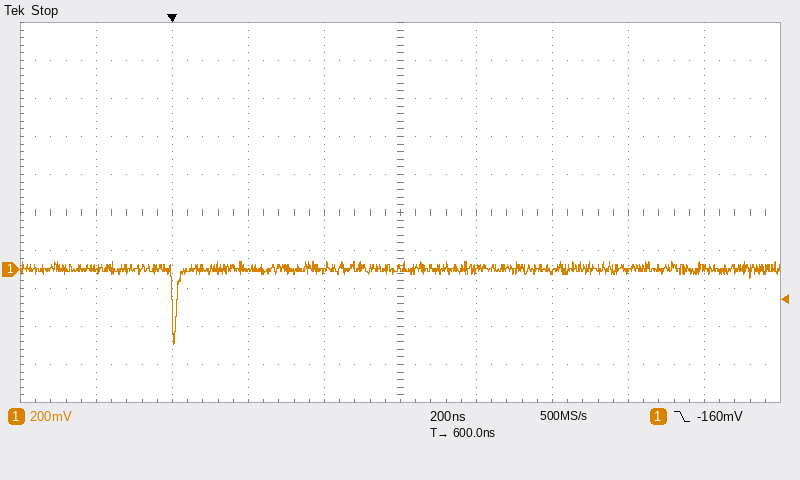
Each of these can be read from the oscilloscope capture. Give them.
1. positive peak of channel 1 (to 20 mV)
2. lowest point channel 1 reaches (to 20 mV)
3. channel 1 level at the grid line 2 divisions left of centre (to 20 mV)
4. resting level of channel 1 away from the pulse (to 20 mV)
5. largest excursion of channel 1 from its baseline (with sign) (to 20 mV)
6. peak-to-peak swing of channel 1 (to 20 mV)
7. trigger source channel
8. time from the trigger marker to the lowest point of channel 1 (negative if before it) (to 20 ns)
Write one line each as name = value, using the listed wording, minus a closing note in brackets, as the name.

positive peak of channel 1 = 40 mV
lowest point channel 1 reaches = -400 mV
channel 1 level at the grid line 2 divisions left of centre = 0 mV
resting level of channel 1 away from the pulse = 0 mV
largest excursion of channel 1 from its baseline (with sign) = -400 mV
peak-to-peak swing of channel 1 = 440 mV
trigger source channel = channel 1
time from the trigger marker to the lowest point of channel 1 (negative if before it) = 0 ns
